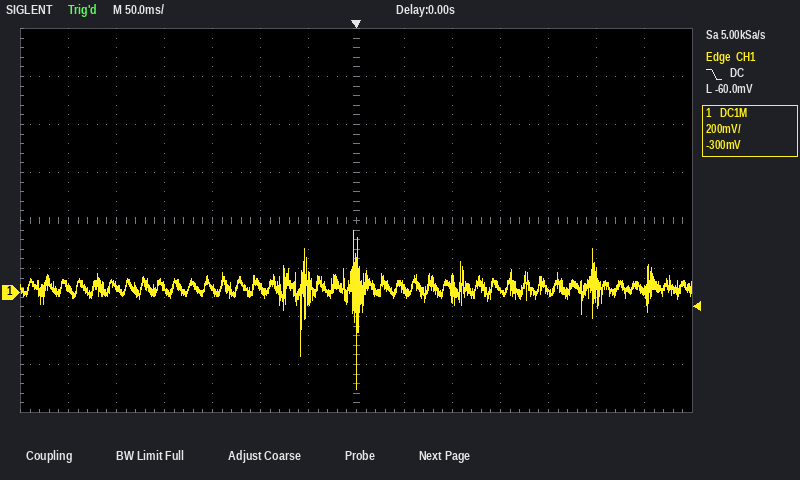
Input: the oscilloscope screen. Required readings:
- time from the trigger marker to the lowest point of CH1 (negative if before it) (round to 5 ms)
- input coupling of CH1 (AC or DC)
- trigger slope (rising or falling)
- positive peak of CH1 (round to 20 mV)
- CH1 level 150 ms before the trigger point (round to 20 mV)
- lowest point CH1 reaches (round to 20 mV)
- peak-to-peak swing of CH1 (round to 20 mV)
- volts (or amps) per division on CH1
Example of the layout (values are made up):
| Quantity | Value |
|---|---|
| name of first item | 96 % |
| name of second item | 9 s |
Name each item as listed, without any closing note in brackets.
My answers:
| Quantity | Value |
|---|---|
| time from the trigger marker to the lowest point of CH1 (negative if before it) | 0 ms |
| input coupling of CH1 | DC |
| trigger slope | falling |
| positive peak of CH1 | 260 mV |
| CH1 level 150 ms before the trigger point | 20 mV |
| lowest point CH1 reaches | -400 mV |
| peak-to-peak swing of CH1 | 660 mV |
| volts (or amps) per division on CH1 | 200 mV |
